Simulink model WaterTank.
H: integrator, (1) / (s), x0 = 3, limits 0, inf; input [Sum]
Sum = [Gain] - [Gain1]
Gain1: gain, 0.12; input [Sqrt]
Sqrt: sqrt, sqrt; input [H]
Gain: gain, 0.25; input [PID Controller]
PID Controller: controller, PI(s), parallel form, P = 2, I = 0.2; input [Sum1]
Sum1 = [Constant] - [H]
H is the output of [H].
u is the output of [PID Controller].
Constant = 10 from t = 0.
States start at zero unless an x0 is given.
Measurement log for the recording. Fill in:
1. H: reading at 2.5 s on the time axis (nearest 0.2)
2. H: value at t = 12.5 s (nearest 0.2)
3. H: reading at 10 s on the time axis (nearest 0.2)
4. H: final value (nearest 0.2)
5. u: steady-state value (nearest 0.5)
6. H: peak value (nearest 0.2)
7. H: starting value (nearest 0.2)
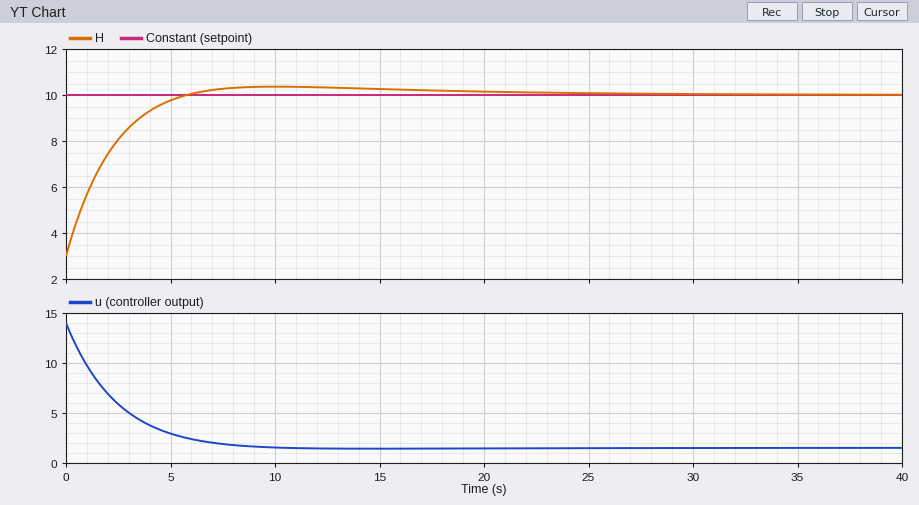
8.0
10.4
10.4
10.0
1.5
10.4
3.0
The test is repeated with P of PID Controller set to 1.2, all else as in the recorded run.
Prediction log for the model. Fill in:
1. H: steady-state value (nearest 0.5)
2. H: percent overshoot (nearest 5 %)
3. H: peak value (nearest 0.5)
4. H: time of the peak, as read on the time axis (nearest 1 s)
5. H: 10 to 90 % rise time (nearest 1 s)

10.0
15 %
11.0
11 s
5 s
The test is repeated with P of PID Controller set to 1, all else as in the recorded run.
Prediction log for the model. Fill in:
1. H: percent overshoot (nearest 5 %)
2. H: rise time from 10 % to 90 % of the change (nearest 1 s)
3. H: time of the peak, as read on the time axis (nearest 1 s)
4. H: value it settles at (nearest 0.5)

20 %
5 s
12 s
10.0
